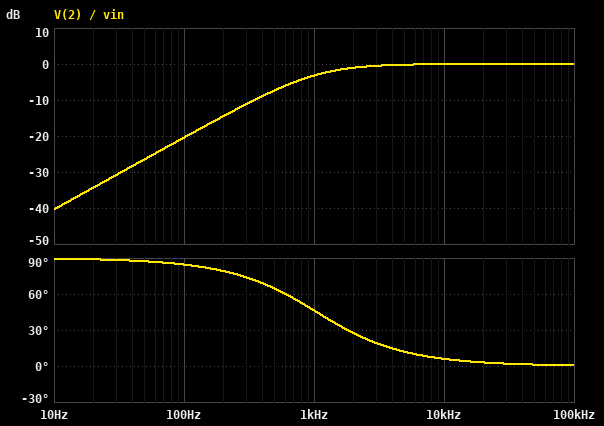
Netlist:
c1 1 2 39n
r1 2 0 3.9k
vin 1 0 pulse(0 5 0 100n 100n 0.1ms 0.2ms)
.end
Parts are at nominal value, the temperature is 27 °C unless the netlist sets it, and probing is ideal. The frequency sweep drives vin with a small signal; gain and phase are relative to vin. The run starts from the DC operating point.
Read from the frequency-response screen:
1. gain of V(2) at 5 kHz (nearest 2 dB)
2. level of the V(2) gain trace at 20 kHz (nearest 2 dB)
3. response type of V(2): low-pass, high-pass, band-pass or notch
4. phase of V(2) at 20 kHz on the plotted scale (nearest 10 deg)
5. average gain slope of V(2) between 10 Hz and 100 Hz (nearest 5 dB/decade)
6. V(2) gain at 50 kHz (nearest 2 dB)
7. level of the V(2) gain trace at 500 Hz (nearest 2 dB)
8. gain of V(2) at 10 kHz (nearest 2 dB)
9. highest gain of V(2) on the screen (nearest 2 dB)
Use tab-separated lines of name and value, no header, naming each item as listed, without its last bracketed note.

gain of V(2) at 5 kHz	0 dB
level of the V(2) gain trace at 20 kHz	0 dB
response type of V(2): low-pass, high-pass, band-pass or notch	high-pass
phase of V(2) at 20 kHz on the plotted scale	0 deg
average gain slope of V(2) between 10 Hz and 100 Hz	20 dB/decade
V(2) gain at 50 kHz	0 dB
level of the V(2) gain trace at 500 Hz	-8 dB
gain of V(2) at 10 kHz	0 dB
highest gain of V(2) on the screen	0 dB
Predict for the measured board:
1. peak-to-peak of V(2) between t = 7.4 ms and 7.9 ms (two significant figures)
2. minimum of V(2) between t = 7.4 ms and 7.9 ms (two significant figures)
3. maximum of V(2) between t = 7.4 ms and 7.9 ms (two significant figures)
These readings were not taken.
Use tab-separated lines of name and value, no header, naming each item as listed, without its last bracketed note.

peak-to-peak of V(2) between t = 7.4 ms and 7.9 ms	6.6 V
minimum of V(2) between t = 7.4 ms and 7.9 ms	-3.3 V
maximum of V(2) between t = 7.4 ms and 7.9 ms	3.3 V
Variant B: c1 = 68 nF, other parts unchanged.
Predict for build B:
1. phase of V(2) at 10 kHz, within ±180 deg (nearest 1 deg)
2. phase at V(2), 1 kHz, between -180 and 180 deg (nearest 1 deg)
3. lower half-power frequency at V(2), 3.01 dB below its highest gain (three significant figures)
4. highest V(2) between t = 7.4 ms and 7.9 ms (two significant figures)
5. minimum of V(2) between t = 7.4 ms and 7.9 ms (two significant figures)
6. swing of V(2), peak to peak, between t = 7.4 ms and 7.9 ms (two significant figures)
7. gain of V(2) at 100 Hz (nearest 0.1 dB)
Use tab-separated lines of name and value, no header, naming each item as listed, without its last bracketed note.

phase of V(2) at 10 kHz, within ±180 deg	3 deg
phase at V(2), 1 kHz, between -180 and 180 deg	31 deg
lower half-power frequency at V(2), 3.01 dB below its highest gain	600 Hz
highest V(2) between t = 7.4 ms and 7.9 ms	3.0 V
minimum of V(2) between t = 7.4 ms and 7.9 ms	-3.0 V
swing of V(2), peak to peak, between t = 7.4 ms and 7.9 ms	5.9 V
gain of V(2) at 100 Hz	-15.7 dB
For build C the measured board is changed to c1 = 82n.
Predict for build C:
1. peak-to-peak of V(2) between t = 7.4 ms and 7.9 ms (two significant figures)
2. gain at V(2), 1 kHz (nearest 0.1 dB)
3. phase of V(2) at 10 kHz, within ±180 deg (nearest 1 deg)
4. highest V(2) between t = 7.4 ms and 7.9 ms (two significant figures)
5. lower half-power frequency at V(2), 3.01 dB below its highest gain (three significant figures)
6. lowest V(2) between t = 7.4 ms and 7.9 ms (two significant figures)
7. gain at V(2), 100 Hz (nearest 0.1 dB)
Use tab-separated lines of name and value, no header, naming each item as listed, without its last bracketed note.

peak-to-peak of V(2) between t = 7.4 ms and 7.9 ms	5.8 V
gain at V(2), 1 kHz	-1.0 dB
phase of V(2) at 10 kHz, within ±180 deg	3 deg
highest V(2) between t = 7.4 ms and 7.9 ms	2.9 V
lower half-power frequency at V(2), 3.01 dB below its highest gain	498 Hz
lowest V(2) between t = 7.4 ms and 7.9 ms	-2.9 V
gain at V(2), 100 Hz	-14.1 dB
